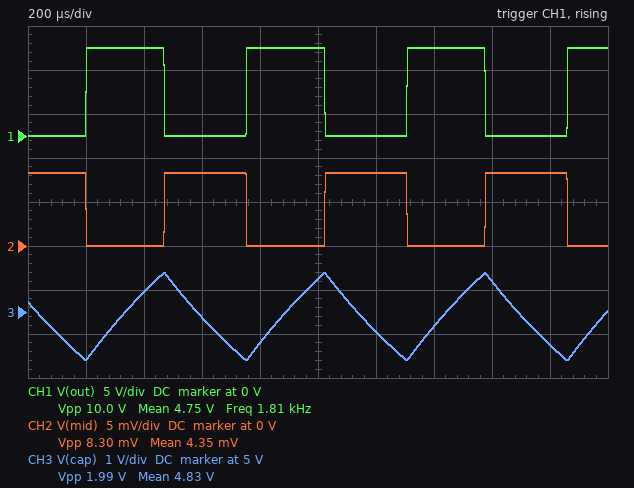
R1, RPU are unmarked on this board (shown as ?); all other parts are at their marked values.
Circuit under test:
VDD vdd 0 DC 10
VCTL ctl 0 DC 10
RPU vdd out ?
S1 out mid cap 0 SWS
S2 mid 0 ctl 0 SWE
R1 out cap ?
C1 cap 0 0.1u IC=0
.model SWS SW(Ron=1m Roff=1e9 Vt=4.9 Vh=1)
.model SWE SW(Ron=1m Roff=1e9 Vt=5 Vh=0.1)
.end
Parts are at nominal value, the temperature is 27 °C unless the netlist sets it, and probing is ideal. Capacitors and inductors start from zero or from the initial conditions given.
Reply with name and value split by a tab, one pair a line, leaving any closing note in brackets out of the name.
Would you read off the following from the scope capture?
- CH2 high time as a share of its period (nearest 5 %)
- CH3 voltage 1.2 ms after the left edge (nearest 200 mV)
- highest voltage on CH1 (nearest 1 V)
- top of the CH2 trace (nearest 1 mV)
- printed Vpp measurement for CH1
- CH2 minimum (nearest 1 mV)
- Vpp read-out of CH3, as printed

CH2 high time as a share of its period	50 %
CH3 voltage 1.2 ms after the left edge	4.6 V
highest voltage on CH1	10 V
top of the CH2 trace	8 mV
printed Vpp measurement for CH1	10.0 V
CH2 minimum	0 V
Vpp read-out of CH3, as printed	1.99 V
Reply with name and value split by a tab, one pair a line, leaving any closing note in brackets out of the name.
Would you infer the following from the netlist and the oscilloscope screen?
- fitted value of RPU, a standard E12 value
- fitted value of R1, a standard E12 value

fitted value of RPU, a standard E12 value	1.2 Ω
fitted value of R1, a standard E12 value	6.8 kΩ
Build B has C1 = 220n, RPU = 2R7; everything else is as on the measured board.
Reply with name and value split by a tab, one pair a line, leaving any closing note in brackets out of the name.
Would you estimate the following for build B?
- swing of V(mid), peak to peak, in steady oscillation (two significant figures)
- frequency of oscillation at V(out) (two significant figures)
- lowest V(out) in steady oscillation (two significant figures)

swing of V(mid), peak to peak, in steady oscillation	3.7 mV
frequency of oscillation at V(out)	820 Hz
lowest V(out) in steady oscillation	7.4 mV
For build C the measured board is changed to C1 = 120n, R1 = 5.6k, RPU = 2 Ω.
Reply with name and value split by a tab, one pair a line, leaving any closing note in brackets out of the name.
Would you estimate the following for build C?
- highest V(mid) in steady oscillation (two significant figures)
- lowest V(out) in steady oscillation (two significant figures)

highest V(mid) in steady oscillation	5.0 mV
lowest V(out) in steady oscillation	10 mV
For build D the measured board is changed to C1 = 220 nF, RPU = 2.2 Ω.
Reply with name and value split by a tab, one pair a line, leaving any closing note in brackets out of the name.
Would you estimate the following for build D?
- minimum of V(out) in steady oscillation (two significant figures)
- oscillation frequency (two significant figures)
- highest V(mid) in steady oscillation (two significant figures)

minimum of V(out) in steady oscillation	9.1 mV
oscillation frequency	820 Hz
highest V(mid) in steady oscillation	4.5 mV
